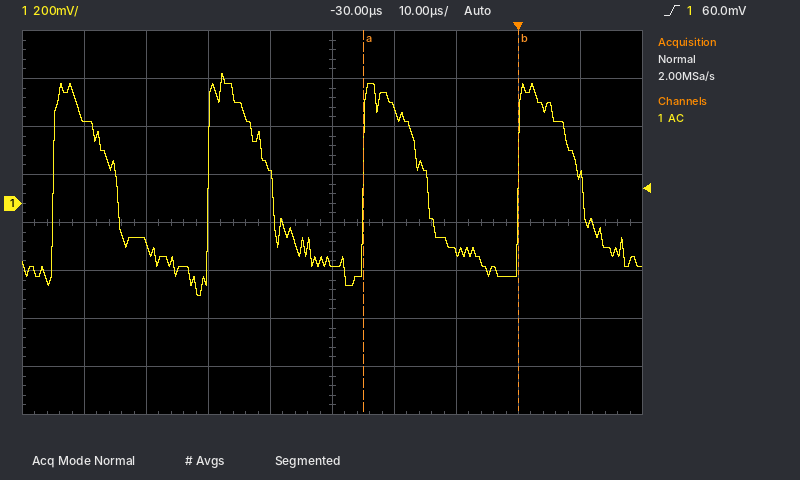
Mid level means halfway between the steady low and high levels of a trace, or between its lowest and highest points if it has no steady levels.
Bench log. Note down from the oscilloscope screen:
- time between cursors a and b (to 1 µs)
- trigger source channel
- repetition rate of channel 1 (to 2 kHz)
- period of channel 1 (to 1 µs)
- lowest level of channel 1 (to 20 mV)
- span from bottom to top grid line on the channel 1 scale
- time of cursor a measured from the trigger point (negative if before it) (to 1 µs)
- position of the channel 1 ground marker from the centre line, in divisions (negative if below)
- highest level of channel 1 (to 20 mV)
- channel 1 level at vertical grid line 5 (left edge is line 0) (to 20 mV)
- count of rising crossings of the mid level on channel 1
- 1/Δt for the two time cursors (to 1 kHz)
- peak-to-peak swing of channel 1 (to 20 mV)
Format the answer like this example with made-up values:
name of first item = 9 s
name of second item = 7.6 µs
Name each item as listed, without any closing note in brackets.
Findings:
time between cursors a and b = 25 µs
trigger source channel = channel 1
repetition rate of channel 1 = 40 kHz
period of channel 1 = 25 µs
lowest level of channel 1 = -380 mV
span from bottom to top grid line on the channel 1 scale = 1.6 V
time of cursor a measured from the trigger point (negative if before it) = -25 µs
position of the channel 1 ground marker from the centre line, in divisions = +0.4 div
highest level of channel 1 = 540 mV
channel 1 level at vertical grid line 5 (left edge is line 0) = -260 mV
count of rising crossings of the mid level on channel 1 = 4
1/Δt for the two time cursors = 40 kHz
peak-to-peak swing of channel 1 = 920 mV
